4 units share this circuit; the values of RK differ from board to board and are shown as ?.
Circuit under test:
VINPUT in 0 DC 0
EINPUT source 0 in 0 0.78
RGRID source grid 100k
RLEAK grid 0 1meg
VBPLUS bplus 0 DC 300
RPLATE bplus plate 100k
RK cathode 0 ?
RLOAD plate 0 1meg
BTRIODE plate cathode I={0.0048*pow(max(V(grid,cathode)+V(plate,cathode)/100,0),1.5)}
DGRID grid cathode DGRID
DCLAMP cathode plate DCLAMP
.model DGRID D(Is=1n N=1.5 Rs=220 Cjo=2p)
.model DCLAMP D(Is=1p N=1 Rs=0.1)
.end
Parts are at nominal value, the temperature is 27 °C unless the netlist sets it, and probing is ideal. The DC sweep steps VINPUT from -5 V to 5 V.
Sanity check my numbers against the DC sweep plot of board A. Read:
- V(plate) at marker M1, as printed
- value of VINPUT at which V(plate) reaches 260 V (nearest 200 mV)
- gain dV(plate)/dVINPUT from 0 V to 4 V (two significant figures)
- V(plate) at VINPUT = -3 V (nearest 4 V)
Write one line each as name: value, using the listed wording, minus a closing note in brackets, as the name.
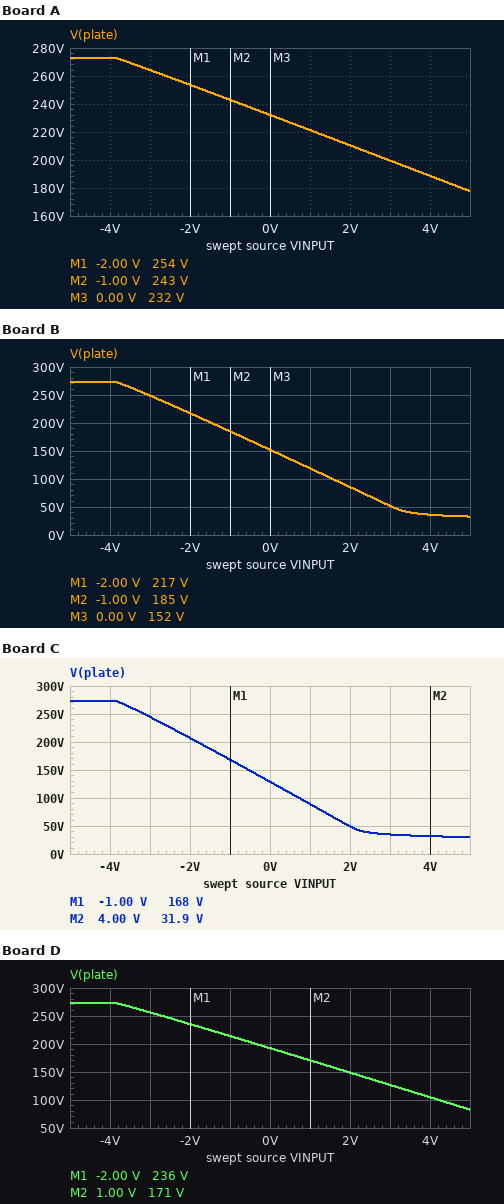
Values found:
V(plate) at marker M1, as printed: 254 V
value of VINPUT at which V(plate) reaches 260 V: -2.6 V
gain dV(plate)/dVINPUT from 0 V to 4 V: -11 V/V
V(plate) at VINPUT = -3 V: 264 V
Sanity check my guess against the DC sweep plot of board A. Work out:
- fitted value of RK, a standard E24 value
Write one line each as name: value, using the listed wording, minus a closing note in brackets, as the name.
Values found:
fitted value of RK, a standard E24 value: 4.7 kΩ
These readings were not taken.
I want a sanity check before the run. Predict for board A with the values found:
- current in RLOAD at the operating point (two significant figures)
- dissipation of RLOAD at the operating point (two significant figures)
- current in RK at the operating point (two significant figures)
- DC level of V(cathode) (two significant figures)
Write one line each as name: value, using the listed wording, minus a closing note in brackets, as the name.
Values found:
current in RLOAD at the operating point: 230 µA
dissipation of RLOAD at the operating point: 54 mW
current in RK at the operating point: 450 µA
DC level of V(cathode): 2.1 V
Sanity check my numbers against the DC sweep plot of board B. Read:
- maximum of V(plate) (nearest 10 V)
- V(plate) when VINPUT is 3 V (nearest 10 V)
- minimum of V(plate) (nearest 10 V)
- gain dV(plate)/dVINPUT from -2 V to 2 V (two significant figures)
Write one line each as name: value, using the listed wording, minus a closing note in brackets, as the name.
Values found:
maximum of V(plate): 270 V
V(plate) when VINPUT is 3 V: 50 V
minimum of V(plate): 30 V
gain dV(plate)/dVINPUT from -2 V to 2 V: -33 V/V
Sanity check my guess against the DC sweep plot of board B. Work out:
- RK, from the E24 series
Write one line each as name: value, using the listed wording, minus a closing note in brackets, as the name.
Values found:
RK, from the E24 series: 820 Ω
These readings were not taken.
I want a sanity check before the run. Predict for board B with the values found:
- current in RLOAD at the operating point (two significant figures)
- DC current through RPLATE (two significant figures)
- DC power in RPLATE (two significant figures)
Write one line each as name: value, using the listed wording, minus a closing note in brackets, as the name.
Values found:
current in RLOAD at the operating point: 150 µA
DC current through RPLATE: 1.5 mA
DC power in RPLATE: 220 mW
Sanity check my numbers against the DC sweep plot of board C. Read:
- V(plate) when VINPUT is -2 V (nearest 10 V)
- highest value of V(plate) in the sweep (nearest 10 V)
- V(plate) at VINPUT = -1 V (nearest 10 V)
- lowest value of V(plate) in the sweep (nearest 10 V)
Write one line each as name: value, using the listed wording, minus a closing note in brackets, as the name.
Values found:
V(plate) when VINPUT is -2 V: 210 V
highest value of V(plate) in the sweep: 270 V
V(plate) at VINPUT = -1 V: 170 V
lowest value of V(plate) in the sweep: 30 V
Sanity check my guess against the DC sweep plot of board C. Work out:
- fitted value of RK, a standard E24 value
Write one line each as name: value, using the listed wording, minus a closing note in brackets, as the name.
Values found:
fitted value of RK, a standard E24 value: 510 Ω
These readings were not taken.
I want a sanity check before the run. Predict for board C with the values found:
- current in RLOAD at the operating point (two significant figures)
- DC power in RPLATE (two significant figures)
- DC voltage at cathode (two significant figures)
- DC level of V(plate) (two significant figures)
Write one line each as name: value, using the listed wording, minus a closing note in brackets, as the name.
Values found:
current in RLOAD at the operating point: 130 µA
DC power in RPLATE: 290 mW
DC voltage at cathode: 810 mV
DC level of V(plate): 130 V
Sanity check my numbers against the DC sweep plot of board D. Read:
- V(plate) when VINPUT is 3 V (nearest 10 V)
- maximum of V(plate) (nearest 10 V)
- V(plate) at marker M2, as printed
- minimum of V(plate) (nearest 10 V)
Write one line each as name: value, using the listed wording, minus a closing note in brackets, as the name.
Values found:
V(plate) when VINPUT is 3 V: 130 V
maximum of V(plate): 270 V
V(plate) at marker M2, as printed: 171 V
minimum of V(plate): 80 V
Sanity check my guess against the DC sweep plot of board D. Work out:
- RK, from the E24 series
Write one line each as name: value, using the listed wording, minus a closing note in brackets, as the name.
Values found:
RK, from the E24 series: 1.8 kΩ
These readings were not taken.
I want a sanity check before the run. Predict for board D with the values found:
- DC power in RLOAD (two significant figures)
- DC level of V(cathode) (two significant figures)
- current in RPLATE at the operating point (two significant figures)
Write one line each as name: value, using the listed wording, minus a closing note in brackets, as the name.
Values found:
DC power in RLOAD: 37 mW
DC level of V(cathode): 1.6 V
current in RPLATE at the operating point: 1.1 mA
